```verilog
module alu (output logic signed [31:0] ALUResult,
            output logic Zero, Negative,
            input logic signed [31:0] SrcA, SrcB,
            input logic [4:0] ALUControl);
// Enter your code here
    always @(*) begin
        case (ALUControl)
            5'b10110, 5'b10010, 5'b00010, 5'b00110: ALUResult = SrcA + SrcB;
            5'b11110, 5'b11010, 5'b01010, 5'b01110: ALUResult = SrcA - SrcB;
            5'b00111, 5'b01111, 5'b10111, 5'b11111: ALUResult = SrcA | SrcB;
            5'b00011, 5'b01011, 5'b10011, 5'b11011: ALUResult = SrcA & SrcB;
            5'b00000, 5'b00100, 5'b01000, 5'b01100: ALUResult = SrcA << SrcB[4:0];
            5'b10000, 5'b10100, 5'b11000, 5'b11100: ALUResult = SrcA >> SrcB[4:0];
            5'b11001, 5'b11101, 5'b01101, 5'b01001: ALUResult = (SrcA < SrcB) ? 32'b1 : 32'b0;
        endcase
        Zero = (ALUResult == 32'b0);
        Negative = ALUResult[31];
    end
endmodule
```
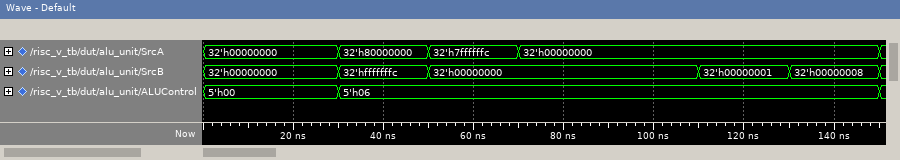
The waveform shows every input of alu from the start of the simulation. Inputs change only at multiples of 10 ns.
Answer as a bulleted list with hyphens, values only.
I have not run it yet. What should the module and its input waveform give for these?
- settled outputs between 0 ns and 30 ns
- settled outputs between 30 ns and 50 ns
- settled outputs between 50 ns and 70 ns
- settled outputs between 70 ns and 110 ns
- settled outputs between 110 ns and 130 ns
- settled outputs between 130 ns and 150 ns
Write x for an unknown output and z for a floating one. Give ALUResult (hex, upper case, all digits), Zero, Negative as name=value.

- ALUResult=00000000, Zero=1, Negative=0
- ALUResult=7FFFFFFC, Zero=0, Negative=0
- ALUResult=7FFFFFFC, Zero=0, Negative=0
- ALUResult=00000000, Zero=1, Negative=0
- ALUResult=00000001, Zero=0, Negative=0
- ALUResult=00000008, Zero=0, Negative=0
